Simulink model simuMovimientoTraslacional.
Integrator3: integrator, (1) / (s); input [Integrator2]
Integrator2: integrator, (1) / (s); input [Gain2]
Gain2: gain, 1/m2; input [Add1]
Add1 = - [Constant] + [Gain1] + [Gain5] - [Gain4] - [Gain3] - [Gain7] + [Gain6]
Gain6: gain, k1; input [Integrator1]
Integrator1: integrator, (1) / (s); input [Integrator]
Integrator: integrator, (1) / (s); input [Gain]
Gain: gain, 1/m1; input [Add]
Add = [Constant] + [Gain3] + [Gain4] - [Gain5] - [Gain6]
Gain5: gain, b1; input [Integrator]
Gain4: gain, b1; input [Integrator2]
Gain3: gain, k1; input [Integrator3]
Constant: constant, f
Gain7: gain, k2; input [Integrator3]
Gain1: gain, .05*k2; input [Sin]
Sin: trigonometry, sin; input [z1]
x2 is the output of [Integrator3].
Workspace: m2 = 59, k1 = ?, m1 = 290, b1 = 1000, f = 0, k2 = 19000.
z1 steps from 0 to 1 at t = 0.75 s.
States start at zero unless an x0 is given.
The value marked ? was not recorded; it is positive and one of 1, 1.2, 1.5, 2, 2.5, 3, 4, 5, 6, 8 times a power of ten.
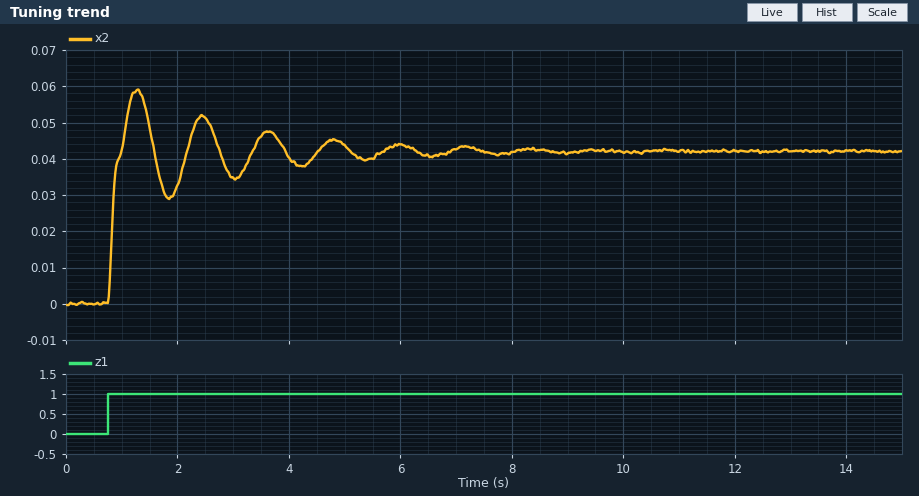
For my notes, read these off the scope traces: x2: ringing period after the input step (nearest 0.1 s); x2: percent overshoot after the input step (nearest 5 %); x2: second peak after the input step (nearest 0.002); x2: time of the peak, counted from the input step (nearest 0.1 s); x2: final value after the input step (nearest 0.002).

1.2 s
40 %
0.052
0.5 s
0.042
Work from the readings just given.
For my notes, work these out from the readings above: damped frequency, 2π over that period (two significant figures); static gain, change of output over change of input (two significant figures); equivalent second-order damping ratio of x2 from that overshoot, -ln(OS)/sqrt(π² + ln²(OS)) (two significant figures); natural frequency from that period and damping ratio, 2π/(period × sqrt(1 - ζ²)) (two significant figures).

5.2 rad/s
0.042
0.28
5.5 rad/s
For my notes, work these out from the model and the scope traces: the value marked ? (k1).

15000
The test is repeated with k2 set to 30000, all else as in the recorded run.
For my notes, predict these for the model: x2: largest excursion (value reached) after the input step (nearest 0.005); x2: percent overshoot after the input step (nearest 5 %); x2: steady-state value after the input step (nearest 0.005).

0.055
30 %
0.040
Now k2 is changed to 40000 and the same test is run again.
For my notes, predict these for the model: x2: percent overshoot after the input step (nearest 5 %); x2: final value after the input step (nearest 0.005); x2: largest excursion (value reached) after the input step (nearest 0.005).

25 %
0.040
0.050
